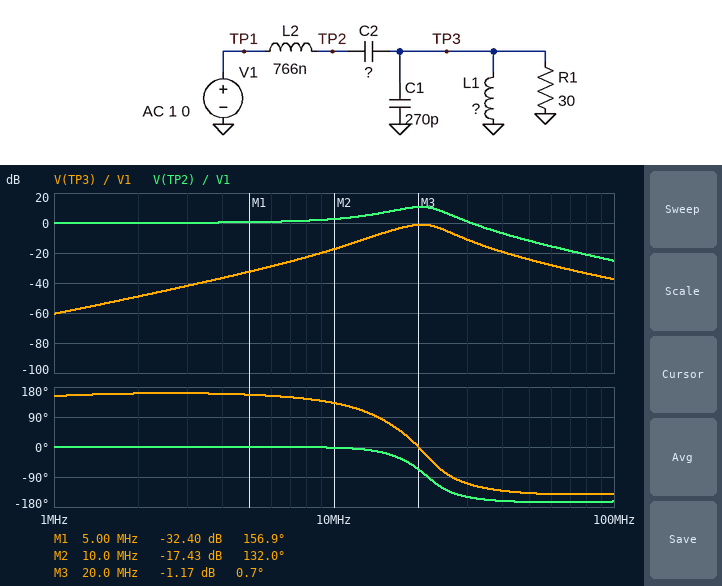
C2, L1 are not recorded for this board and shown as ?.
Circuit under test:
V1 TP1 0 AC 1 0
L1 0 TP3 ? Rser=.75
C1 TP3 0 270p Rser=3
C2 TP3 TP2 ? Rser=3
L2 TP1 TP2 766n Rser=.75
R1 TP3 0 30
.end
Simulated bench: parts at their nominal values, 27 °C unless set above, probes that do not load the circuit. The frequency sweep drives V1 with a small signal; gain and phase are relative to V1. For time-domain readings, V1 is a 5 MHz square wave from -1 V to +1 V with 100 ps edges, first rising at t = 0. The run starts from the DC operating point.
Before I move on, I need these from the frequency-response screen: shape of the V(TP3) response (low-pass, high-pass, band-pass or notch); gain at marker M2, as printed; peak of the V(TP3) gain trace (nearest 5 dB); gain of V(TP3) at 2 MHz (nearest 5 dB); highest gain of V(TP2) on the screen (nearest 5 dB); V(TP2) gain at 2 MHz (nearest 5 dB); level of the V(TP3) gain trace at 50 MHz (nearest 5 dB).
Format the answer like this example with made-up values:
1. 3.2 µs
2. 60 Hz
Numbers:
1. band-pass
2. -17.43 dB
3. 0 dB
4. -50 dB
5. 10 dB
6. 0 dB
7. -25 dB
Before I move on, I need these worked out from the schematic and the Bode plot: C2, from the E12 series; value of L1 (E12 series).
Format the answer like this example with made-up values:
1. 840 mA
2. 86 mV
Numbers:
1. 82 pF
2. 270 nH
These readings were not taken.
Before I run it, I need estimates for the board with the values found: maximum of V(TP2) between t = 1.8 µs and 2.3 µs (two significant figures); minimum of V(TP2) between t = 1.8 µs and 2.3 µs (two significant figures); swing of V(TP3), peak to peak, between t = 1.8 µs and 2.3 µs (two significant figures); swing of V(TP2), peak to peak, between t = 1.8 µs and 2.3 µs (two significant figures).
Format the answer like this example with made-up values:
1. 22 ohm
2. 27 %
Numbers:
1. 2.4 V
2. -2.4 V
3. 710 mV
4. 4.8 V
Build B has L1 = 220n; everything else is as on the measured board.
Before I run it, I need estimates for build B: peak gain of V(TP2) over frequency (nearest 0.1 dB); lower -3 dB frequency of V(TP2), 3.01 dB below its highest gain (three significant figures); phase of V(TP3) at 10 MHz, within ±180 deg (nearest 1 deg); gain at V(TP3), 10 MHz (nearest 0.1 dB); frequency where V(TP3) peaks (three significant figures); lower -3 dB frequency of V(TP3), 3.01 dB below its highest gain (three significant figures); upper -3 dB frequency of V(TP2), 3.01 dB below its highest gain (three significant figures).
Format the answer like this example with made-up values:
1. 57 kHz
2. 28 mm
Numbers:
1. 10.5 dB
2. 15.1 MHz
3. 140 deg
4. -19.1 dB
5. 19.7 MHz
6. 16.4 MHz
7. 23.7 MHz
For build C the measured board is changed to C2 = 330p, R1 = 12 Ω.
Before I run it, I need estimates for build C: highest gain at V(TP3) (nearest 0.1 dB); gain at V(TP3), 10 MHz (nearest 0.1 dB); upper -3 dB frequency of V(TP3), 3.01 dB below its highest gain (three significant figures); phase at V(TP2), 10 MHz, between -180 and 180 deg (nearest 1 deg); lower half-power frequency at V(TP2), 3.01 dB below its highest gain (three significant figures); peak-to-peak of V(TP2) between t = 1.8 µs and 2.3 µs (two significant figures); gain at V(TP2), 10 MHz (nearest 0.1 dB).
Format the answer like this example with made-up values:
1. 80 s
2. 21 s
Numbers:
1. -2.0 dB
2. -2.5 dB
3. 11.0 MHz
4. -93 deg
5. 7.89 MHz
6. 3.9 V
7. 10.3 dB
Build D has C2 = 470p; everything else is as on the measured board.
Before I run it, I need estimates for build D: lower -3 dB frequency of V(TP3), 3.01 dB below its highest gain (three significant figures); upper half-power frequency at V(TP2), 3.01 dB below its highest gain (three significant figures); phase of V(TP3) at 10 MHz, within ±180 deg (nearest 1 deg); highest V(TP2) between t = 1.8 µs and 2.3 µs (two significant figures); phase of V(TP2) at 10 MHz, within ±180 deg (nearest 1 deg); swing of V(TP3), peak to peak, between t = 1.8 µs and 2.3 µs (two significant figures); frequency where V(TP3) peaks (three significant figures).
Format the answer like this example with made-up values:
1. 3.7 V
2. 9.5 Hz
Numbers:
1. 6.62 MHz
2. 7.82 MHz
3. -12 deg
4. 2.1 V
5. -115 deg
6. 820 mV
7. 7.30 MHz
